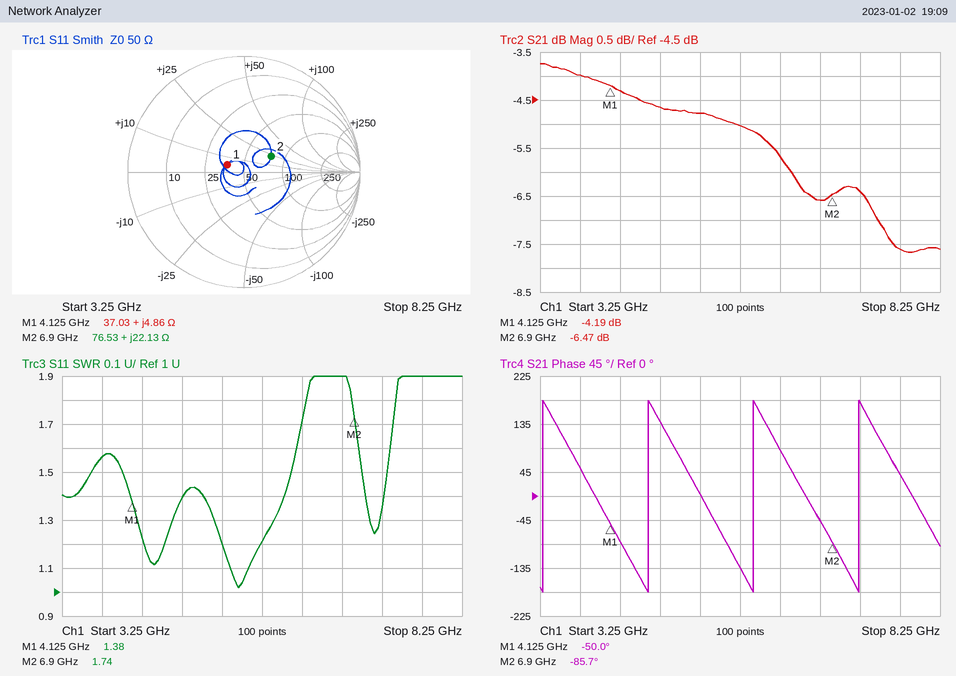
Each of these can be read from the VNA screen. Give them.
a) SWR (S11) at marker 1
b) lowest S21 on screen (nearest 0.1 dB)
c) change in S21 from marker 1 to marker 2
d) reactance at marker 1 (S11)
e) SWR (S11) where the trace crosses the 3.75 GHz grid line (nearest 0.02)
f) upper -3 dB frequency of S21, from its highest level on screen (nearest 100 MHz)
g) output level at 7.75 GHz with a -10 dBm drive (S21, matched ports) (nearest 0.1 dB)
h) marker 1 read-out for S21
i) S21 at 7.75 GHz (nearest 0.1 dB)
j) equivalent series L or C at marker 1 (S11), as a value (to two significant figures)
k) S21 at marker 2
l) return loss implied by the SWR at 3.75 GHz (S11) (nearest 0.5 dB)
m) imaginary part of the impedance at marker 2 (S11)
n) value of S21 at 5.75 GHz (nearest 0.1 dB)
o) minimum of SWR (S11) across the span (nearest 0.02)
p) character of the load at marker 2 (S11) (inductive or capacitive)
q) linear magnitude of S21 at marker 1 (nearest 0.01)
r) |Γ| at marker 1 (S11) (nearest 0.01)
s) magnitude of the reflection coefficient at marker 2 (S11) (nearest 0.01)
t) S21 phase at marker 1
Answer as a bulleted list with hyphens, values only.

- 1.38
- -7.7 dB
- -2.28 dB
- +4.86 Ω
- 1.56
- 7.4 GHz
- -17.6 dBm
- -4.19 dB
- -7.6 dB
- 190 pH
- -6.47 dB
- 13.0 dB
- +22.13 Ω
- -5.0 dB
- 1.02
- inductive
- 0.62
- 0.16
- 0.27
- -50.0°
